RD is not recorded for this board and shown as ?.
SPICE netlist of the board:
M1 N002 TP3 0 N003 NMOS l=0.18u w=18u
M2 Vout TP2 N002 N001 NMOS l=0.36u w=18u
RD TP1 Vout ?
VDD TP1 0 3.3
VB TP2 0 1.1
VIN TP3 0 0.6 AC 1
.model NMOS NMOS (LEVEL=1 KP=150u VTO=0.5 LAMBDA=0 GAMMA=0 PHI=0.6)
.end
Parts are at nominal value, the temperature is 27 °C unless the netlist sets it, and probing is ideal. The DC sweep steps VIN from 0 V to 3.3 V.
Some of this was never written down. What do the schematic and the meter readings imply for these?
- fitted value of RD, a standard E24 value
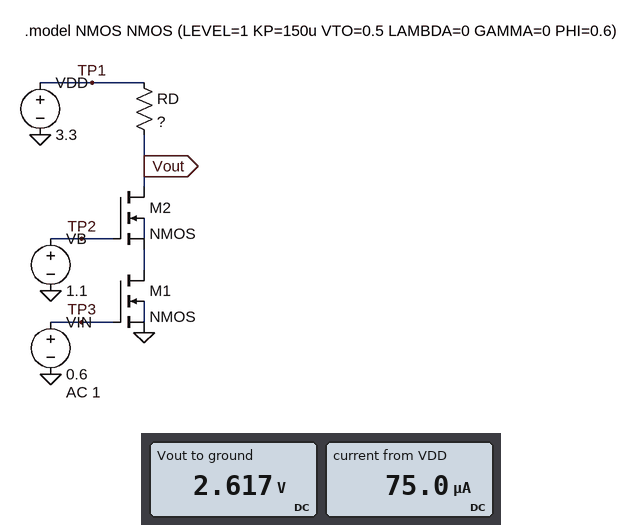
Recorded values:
9.1 kΩ
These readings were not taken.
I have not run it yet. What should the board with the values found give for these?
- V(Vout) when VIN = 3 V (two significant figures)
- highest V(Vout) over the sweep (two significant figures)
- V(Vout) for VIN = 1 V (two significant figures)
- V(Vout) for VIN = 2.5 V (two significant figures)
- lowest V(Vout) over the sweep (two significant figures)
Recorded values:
95 mV
3.3 V
140 mV
98 mV
94 mV
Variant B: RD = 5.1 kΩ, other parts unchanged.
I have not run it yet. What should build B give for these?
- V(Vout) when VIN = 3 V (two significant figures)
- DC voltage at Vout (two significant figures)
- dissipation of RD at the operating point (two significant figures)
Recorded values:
180 mV
2.9 V
29 µW
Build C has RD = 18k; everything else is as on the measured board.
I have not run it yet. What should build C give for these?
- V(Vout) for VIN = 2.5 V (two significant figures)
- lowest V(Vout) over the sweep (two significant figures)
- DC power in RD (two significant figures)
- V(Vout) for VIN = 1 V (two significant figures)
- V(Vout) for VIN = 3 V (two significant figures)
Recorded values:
48 mV
46 mV
100 µW
68 mV
47 mV
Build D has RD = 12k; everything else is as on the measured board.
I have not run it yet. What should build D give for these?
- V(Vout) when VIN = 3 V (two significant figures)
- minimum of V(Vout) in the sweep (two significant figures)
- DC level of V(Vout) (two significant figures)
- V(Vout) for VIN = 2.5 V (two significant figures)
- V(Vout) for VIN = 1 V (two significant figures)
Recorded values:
71 mV
70 mV
2.4 V
73 mV
100 mV
